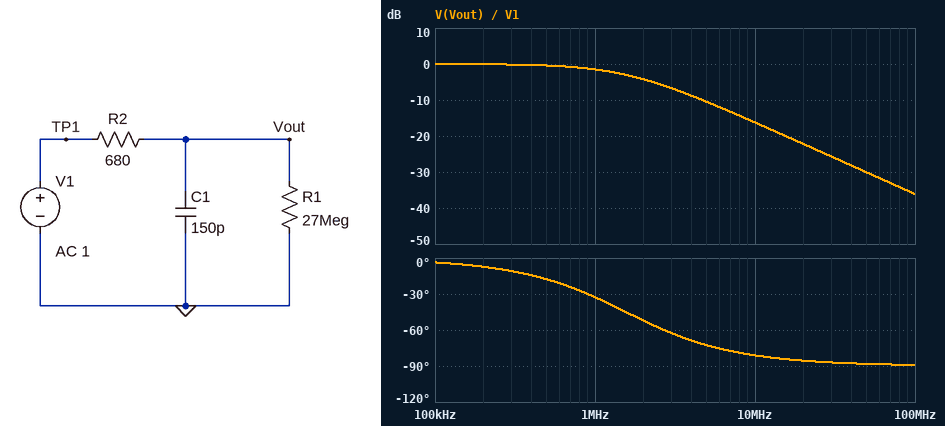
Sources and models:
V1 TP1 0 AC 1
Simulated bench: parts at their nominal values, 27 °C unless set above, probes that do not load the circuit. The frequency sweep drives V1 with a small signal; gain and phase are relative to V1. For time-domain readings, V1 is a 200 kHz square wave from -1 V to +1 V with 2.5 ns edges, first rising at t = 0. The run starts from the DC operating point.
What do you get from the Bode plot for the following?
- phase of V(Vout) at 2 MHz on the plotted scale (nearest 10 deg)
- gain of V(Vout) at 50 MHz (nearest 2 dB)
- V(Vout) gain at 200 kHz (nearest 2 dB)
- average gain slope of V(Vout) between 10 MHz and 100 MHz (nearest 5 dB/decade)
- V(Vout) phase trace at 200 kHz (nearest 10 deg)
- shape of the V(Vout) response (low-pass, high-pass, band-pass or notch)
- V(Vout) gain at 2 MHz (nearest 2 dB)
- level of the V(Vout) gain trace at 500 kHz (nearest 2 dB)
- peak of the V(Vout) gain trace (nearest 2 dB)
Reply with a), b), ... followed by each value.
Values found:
a) -50 deg
b) -30 dB
c) 0 dB
d) -20 dB/decade
e) -10 deg
f) low-pass
g) -4 dB
h) 0 dB
i) 0 dB
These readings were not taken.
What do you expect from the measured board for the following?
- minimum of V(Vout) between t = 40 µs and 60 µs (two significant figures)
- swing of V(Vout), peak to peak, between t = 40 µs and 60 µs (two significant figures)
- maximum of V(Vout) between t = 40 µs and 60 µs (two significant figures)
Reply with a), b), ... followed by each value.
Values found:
a) -1.0 V
b) 2.0 V
c) 1.0 V
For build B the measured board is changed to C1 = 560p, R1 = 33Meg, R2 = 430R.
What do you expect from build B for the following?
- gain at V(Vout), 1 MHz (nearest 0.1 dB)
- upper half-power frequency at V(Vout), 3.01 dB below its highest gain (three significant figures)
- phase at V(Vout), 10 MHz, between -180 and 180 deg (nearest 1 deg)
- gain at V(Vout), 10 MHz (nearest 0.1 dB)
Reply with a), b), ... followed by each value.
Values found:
a) -5.2 dB
b) 661 kHz
c) -86 deg
d) -23.6 dB
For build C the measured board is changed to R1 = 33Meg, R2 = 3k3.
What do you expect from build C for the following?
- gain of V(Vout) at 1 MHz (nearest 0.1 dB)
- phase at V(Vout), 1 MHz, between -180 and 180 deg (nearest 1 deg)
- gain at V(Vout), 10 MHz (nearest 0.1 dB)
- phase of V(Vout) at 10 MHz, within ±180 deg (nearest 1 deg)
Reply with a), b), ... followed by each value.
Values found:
a) -10.3 dB
b) -72 deg
c) -29.9 dB
d) -88 deg
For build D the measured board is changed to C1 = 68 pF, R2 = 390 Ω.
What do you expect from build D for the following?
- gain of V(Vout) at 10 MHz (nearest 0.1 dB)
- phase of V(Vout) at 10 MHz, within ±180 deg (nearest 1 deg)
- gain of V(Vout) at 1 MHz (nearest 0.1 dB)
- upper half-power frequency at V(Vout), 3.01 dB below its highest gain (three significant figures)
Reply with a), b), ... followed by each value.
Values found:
a) -5.8 dB
b) -59 deg
c) -0.1 dB
d) 6.00 MHz
